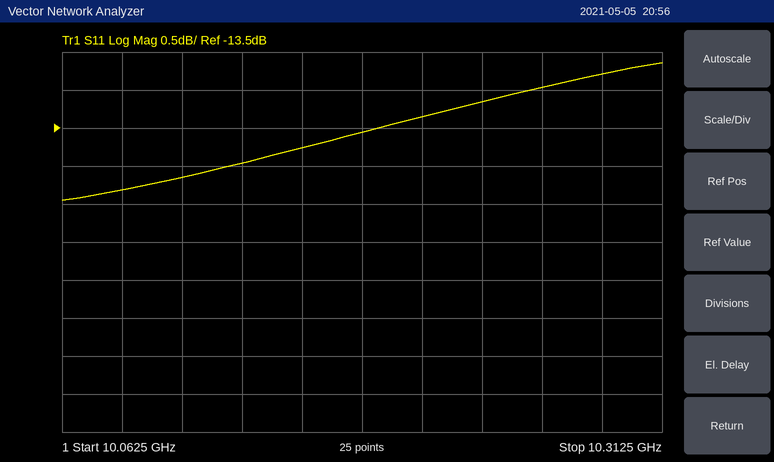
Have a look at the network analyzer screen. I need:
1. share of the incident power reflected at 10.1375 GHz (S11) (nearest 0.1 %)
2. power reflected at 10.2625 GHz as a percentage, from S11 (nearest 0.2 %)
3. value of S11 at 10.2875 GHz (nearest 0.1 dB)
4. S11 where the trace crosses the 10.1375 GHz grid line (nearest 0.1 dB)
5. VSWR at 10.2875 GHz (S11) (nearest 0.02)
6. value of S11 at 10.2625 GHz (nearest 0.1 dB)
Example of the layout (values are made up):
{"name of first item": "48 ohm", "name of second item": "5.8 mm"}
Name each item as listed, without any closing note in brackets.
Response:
{"share of the incident power reflected at 10.1375 GHz (S11)": "4.0 %", "power reflected at 10.2625 GHz as a percentage, from S11": "5.0 %", "value of S11 at 10.2875 GHz": "-12.8 dB", "S11 where the trace crosses the 10.1375 GHz grid line": "-14.0 dB", "VSWR at 10.2875 GHz (S11)": "1.60", "value of S11 at 10.2625 GHz": "-13.0 dB"}
